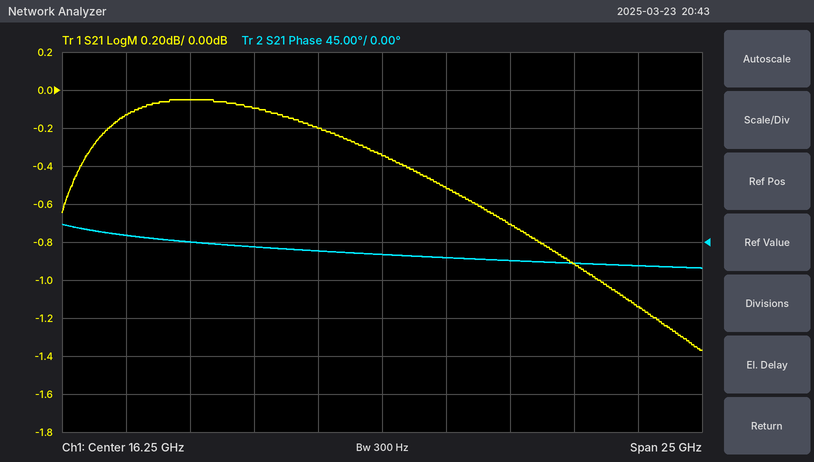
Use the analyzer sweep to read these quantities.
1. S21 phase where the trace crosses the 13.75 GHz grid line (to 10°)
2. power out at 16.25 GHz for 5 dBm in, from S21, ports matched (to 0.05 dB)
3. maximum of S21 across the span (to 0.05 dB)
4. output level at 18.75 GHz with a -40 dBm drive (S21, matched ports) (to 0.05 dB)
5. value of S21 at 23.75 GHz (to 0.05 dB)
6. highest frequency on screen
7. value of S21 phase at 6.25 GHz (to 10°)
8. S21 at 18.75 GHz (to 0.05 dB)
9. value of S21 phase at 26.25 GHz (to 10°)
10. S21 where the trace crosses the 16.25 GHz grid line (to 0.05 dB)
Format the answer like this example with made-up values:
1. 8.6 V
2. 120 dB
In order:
1. -10°
2. 4.65 dBm
3. -0.05 dB
4. -40.50 dBm
5. -0.90 dB
6. 28.75 GHz
7. 10°
8. -0.50 dB
9. -30°
10. -0.35 dB
